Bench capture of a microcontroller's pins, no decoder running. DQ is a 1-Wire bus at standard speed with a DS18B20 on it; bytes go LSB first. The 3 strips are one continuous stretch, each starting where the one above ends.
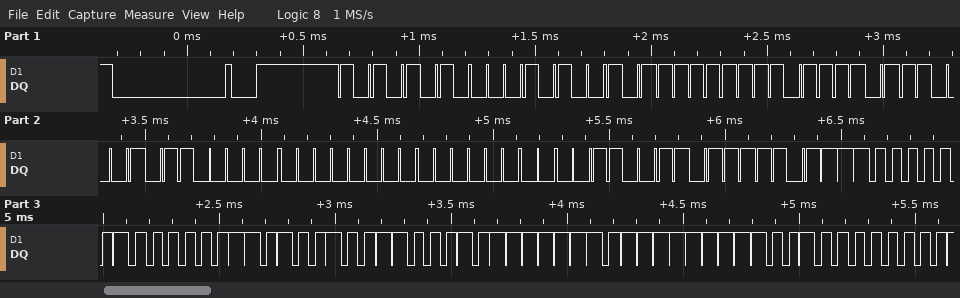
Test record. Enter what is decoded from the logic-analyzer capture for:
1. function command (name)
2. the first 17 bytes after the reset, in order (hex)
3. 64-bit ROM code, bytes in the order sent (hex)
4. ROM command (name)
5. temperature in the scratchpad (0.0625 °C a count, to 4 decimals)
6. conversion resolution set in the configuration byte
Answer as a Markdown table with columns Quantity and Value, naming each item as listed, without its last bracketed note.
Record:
| Quantity | Value |
|---|---|
| function command | Read Scratchpad |
| the first 17 bytes after the reset, in order | 55 28 FD F7 8E 06 00 00 CC BE 07 02 4B 46 7F FF 09 |
| 64-bit ROM code, bytes in the order sent | 28 FD F7 8E 06 00 00 CC |
| ROM command | Match ROM |
| temperature in the scratchpad | 32.4375 °C |
| conversion resolution set in the configuration byte | 12 bits |
